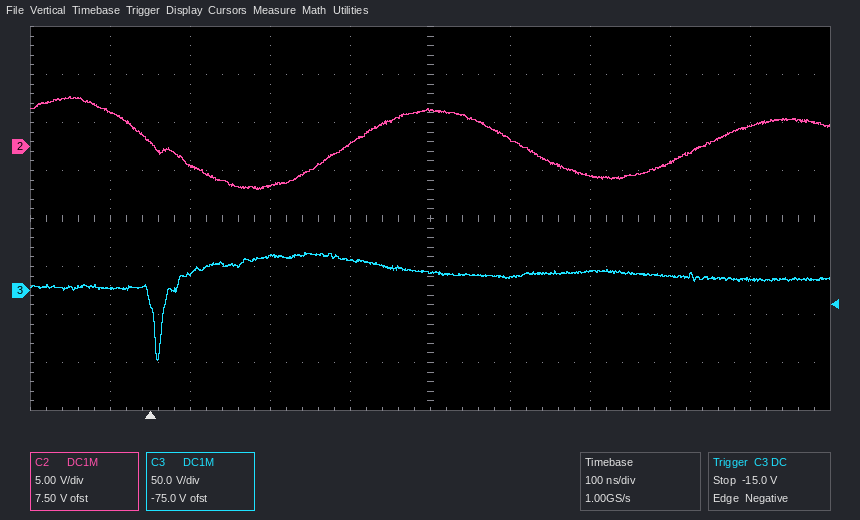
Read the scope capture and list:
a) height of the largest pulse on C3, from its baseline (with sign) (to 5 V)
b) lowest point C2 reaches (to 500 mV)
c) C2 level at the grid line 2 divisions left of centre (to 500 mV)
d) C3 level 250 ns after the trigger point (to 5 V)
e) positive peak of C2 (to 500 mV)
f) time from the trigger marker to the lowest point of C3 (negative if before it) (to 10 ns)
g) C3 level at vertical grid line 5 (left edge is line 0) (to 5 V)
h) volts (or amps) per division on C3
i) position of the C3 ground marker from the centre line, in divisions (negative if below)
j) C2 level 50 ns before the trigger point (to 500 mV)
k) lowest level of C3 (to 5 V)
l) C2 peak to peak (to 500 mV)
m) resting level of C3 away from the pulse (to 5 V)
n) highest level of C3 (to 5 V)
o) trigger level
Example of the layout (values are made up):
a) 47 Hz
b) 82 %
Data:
a) -90 V
b) -4.5 V
c) -4.0 V
d) 30 V
e) 5.0 V
f) +10 ns
g) 20 V
h) 50 V
i) -1.5 div
j) 3.5 V
k) -75 V
l) 9.5 V
m) 15 V
n) 40 V
o) -15.0 V
